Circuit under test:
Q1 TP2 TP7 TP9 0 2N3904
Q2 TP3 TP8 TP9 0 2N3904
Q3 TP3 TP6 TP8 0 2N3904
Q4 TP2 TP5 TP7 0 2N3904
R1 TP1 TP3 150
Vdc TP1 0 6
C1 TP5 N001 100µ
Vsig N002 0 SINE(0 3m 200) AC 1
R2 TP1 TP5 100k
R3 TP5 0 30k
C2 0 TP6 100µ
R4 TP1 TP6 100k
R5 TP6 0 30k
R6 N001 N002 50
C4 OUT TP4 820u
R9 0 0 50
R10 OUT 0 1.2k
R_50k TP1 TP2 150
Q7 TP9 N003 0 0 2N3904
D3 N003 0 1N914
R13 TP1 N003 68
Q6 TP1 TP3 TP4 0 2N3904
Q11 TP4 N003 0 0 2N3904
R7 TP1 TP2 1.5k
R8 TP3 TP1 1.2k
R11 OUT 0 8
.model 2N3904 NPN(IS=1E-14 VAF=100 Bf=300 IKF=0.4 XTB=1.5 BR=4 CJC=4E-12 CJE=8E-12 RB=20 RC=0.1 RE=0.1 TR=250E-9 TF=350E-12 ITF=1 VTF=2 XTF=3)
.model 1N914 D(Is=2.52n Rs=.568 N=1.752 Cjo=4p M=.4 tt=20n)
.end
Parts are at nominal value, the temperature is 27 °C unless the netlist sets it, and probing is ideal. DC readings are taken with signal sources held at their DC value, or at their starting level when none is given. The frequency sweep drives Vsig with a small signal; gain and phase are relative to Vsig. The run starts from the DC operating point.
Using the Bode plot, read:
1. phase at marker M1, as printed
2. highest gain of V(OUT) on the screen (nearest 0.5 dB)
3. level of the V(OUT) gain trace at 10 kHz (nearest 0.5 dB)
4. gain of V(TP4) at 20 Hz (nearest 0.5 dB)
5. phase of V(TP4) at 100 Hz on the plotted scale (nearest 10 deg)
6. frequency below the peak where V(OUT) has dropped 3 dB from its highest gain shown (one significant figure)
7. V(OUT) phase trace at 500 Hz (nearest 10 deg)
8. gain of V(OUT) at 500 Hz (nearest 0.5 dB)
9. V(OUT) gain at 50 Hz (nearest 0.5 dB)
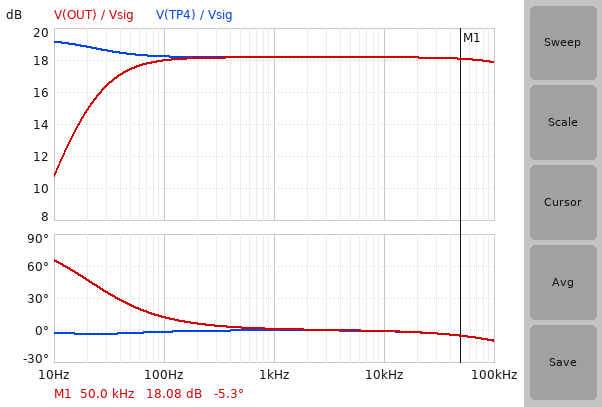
-5.3 deg
18.0 dB
18.0 dB
19.0 dB
0 deg
20 Hz
0 deg
18.0 dB
17.5 dB
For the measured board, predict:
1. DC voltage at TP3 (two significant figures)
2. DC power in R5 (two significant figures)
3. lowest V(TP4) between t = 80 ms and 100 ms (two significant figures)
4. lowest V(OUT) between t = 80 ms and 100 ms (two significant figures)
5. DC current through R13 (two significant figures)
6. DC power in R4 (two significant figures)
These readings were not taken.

3.1 V
63 µW
2.3 V
-24 mV
76 mA
210 µW
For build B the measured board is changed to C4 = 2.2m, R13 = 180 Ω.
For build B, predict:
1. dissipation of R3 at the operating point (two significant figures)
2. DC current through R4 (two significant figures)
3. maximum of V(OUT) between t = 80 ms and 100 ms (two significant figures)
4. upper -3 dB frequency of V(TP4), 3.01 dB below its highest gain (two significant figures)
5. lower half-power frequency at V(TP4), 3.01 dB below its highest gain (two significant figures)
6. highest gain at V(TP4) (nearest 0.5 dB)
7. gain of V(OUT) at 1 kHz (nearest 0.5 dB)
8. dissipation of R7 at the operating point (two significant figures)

64 µW
46 µA
25 mV
320 kHz
73 mHz
20.0 dB
18.5 dB
2.0 mW
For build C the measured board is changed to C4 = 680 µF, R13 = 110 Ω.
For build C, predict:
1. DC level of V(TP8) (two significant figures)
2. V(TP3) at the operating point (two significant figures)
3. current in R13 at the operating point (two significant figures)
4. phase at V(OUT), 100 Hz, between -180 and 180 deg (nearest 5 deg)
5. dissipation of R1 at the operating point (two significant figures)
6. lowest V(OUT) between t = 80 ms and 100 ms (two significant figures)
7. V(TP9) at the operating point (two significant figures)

800 mV
3.6 V
47 mA
15 deg
38 mW
-25 mV
66 mV
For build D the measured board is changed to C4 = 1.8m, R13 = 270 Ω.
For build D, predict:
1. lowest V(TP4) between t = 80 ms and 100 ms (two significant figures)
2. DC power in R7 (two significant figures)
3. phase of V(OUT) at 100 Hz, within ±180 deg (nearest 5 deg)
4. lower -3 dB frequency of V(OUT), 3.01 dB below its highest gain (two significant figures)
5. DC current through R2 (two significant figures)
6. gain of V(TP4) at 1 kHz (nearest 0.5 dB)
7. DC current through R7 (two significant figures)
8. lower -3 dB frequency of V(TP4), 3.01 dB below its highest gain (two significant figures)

4.3 V
670 µW
5 deg
8.6 Hz
46 µA
16.0 dB
670 µA
71 mHz
